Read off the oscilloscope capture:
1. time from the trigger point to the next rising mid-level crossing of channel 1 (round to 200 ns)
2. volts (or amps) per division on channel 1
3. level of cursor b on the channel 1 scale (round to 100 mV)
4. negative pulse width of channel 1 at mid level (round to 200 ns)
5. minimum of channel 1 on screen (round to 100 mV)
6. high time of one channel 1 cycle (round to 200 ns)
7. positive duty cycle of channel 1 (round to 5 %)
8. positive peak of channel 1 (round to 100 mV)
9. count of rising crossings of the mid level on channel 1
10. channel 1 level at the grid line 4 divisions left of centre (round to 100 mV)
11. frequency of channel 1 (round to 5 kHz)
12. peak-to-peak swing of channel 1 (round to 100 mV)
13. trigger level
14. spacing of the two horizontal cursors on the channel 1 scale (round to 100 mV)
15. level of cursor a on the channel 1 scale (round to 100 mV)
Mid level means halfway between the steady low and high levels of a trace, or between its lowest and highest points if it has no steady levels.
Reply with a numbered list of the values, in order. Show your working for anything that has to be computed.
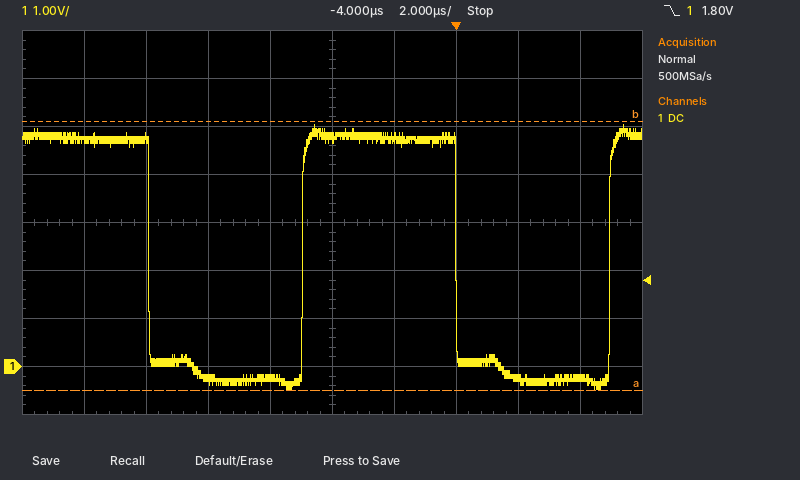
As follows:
1. 5.0 µs
2. 1 V
3. 5.1 V
4. 5.0 µs
5. -500 mV
6. 5.0 µs
7. 50 %
8. 5.0 V
9. 2
10. 4.7 V
11. 100 kHz
12. 5.0 V − (-500 mV) = 5.5 V
13. 1.80 V
14. 5.6 V
15. -500 mV
